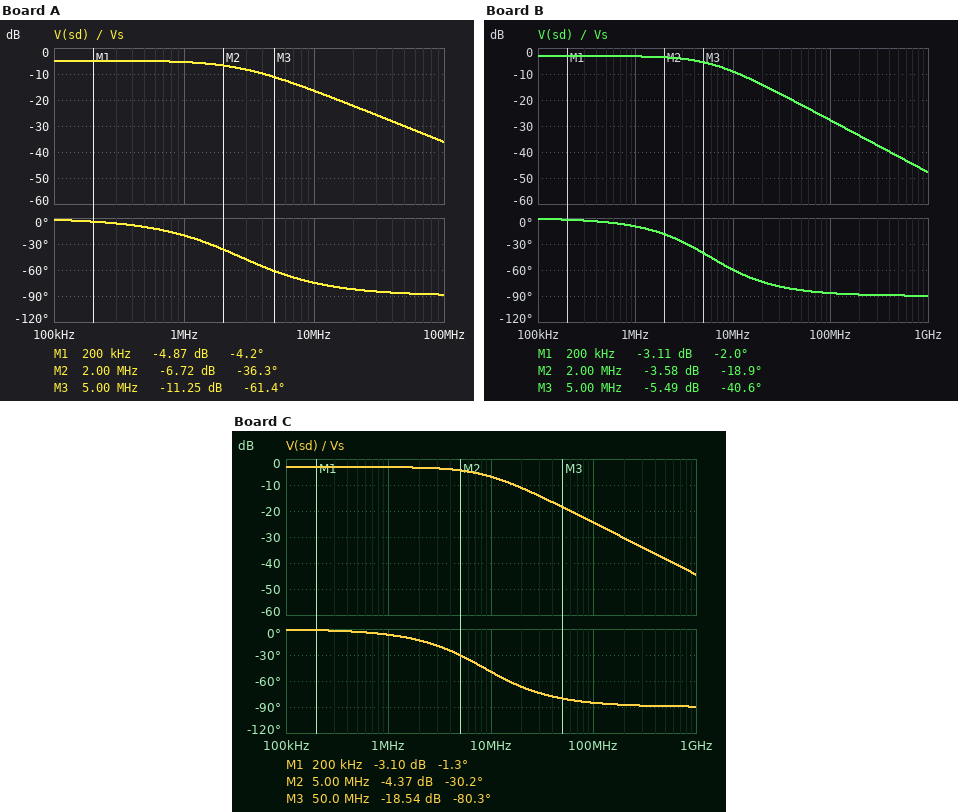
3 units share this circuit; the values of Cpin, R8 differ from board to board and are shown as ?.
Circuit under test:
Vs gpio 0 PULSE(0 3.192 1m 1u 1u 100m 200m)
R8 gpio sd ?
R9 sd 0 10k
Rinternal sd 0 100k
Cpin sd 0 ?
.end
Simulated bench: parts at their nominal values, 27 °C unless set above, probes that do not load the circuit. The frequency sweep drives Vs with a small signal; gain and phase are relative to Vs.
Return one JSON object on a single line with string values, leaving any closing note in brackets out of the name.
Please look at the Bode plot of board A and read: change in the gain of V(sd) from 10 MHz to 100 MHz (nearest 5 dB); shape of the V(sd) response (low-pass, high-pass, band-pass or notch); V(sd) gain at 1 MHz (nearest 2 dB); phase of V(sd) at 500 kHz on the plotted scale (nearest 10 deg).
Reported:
{"change in the gain of V(sd) from 10 MHz to 100 MHz": "-20 dB", "shape of the V(sd) response": "low-pass", "V(sd) gain at 1 MHz": "-6 dB", "phase of V(sd) at 500 kHz on the plotted scale": "-10 deg"}
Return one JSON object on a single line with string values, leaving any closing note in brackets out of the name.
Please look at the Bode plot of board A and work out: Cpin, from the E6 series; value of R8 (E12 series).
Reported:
{"Cpin, from the E6 series": "15 pF", "value of R8": "6.8 kΩ"}
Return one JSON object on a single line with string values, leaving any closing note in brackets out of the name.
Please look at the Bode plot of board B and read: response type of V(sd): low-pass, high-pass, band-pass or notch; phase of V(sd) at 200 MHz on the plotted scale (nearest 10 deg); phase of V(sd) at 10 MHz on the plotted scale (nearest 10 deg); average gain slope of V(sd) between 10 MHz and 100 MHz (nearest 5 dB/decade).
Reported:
{"response type of V(sd): low-pass, high-pass, band-pass or notch": "low-pass", "phase of V(sd) at 200 MHz on the plotted scale": "-90 deg", "phase of V(sd) at 10 MHz on the plotted scale": "-60 deg", "average gain slope of V(sd) between 10 MHz and 100 MHz": "-20 dB/decade"}
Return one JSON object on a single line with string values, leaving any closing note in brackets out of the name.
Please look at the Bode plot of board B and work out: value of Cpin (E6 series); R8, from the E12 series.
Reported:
{"value of Cpin": "10 pF", "R8, from the E12 series": "3.9 kΩ"}
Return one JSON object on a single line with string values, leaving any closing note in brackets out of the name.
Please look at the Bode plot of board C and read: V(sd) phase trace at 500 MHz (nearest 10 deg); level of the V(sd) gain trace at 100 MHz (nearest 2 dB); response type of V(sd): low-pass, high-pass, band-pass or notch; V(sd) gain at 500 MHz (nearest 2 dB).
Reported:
{"V(sd) phase trace at 500 MHz": "-90 deg", "level of the V(sd) gain trace at 100 MHz": "-24 dB", "response type of V(sd): low-pass, high-pass, band-pass or notch": "low-pass", "V(sd) gain at 500 MHz": "-38 dB"}
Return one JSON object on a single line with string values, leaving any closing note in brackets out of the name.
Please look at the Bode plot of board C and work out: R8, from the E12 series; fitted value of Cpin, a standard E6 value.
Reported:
{"R8, from the E12 series": "3.9 kΩ", "fitted value of Cpin, a standard E6 value": "6.8 pF"}
